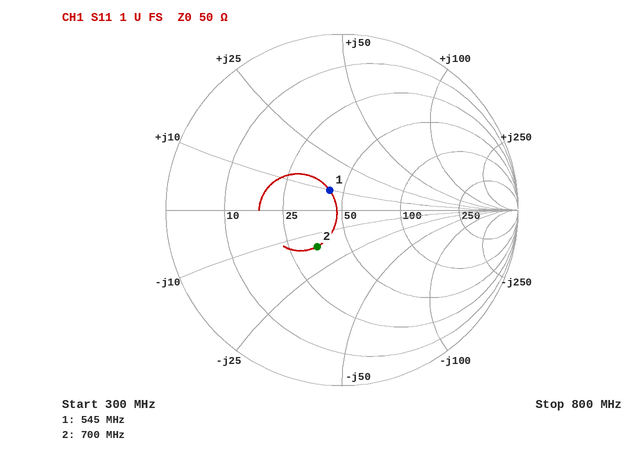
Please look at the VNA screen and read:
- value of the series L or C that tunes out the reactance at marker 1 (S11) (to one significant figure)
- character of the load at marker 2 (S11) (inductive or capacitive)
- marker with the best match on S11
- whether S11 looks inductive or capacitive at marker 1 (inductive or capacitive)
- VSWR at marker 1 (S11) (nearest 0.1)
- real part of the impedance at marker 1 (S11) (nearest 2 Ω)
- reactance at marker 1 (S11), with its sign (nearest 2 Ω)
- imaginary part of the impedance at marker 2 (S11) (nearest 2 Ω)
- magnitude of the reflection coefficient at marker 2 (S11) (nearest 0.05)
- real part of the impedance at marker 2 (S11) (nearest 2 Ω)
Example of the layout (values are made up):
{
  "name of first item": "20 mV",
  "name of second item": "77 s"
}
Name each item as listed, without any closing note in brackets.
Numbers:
{
  "value of the series L or C that tunes out the reactance at marker 1 (S11)": "30 pF",
  "character of the load at marker 2 (S11)": "capacitive",
  "marker with the best match on S11": "marker 1",
  "whether S11 looks inductive or capacitive at marker 1": "inductive",
  "VSWR at marker 1 (S11)": "1.3",
  "real part of the impedance at marker 1 (S11)": "42 Ω",
  "reactance at marker 1 (S11), with its sign": "+10 Ω",
  "imaginary part of the impedance at marker 2 (S11)": "-16 Ω",
  "magnitude of the reflection coefficient at marker 2 (S11)": "0.25",
  "real part of the impedance at marker 2 (S11)": "34 Ω"
}
